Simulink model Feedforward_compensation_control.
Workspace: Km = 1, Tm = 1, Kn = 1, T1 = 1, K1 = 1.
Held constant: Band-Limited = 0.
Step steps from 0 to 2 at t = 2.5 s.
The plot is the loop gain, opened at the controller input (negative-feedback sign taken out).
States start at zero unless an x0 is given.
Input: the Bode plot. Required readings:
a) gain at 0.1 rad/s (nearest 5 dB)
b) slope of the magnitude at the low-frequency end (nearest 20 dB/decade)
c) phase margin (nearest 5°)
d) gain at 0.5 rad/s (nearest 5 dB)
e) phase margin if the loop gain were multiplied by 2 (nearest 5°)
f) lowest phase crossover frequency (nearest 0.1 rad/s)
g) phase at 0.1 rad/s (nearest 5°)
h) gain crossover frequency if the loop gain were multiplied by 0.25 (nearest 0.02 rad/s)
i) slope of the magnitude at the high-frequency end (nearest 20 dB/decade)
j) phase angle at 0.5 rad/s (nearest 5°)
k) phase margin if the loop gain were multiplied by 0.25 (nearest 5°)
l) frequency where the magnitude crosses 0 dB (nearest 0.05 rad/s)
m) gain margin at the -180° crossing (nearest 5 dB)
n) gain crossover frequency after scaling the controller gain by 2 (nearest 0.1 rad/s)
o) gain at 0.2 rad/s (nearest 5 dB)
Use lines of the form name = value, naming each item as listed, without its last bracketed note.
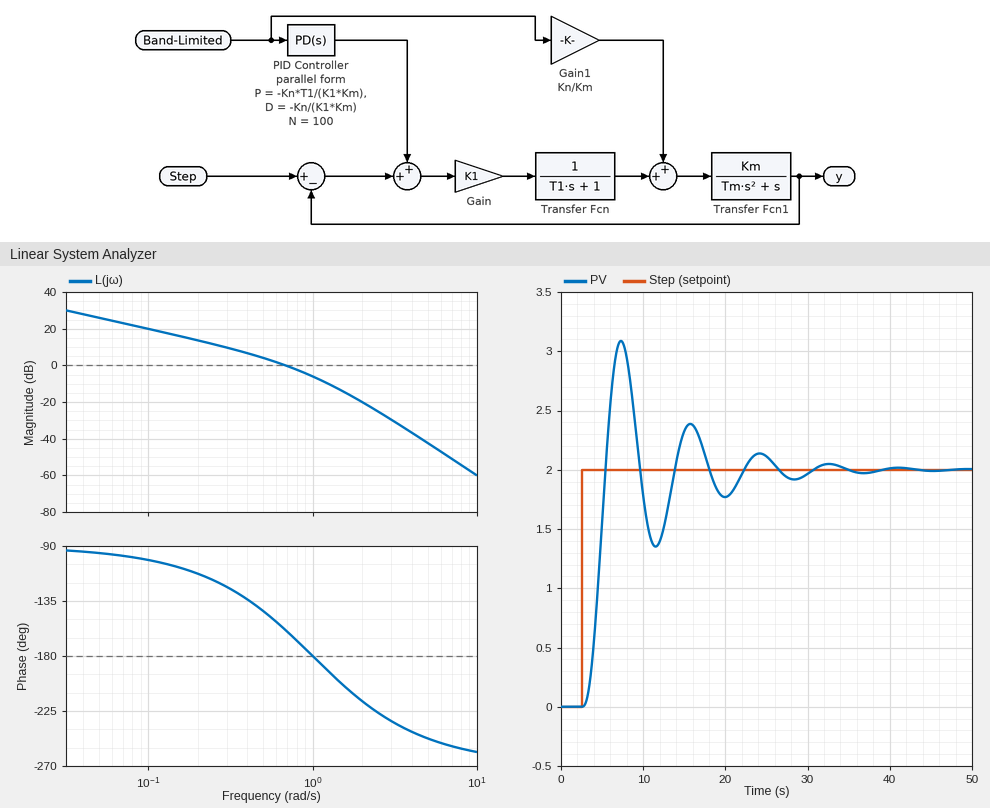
gain at 0.1 rad/s = 20 dB
slope of the magnitude at the low-frequency end = -20 dB/decade
phase margin = 20°
gain at 0.5 rad/s = 5 dB
phase margin if the loop gain were multiplied by 2 = 0°
lowest phase crossover frequency = 1.0 rad/s
phase at 0.1 rad/s = -100°
gain crossover frequency if the loop gain were multiplied by 0.25 = 0.24 rad/s
slope of the magnitude at the high-frequency end = -60 dB/decade
phase angle at 0.5 rad/s = -145°
phase margin if the loop gain were multiplied by 0.25 = 65°
frequency where the magnitude crosses 0 dB = 0.70 rad/s
gain margin at the -180° crossing = 5 dB
gain crossover frequency after scaling the controller gain by 2 = 1.0 rad/s
gain at 0.2 rad/s = 15 dB
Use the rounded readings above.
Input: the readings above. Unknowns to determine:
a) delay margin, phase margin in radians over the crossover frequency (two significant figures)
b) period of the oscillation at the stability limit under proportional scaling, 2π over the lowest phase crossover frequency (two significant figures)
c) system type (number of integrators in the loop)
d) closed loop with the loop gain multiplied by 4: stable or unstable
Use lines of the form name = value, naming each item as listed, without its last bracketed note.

delay margin, phase margin in radians over the crossover frequency = 0.50 s
period of the oscillation at the stability limit under proportional scaling, 2π over the lowest phase crossover frequency = 6.3 s
system type = 1
closed loop with the loop gain multiplied by 4: stable or unstable = unstable
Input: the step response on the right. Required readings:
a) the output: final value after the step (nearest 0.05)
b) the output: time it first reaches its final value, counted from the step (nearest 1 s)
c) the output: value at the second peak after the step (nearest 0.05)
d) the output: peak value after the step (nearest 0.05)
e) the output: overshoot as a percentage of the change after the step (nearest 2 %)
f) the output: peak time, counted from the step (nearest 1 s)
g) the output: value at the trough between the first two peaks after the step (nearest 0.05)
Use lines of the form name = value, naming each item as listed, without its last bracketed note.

the output: final value after the step = 2.00
the output: time it first reaches its final value, counted from the step = 3 s
the output: value at the second peak after the step = 2.40
the output: peak value after the step = 3.10
the output: overshoot as a percentage of the change after the step = 54 %
the output: peak time, counted from the step = 5 s
the output: value at the trough between the first two peaks after the step = 1.35
